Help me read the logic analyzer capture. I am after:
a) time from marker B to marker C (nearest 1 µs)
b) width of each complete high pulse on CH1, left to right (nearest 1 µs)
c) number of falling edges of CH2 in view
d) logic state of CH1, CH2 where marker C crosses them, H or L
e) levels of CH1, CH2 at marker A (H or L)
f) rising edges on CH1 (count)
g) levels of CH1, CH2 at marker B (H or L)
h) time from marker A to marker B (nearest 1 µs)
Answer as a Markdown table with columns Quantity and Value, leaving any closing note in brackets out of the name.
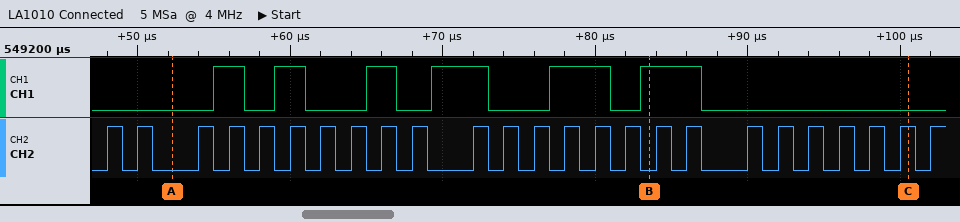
| Quantity | Value |
|---|---|
| time from marker B to marker C | 17 µs |
| width of each complete high pulse on CH1, left to right | 2 µs, 2 µs, 2 µs, 4 µs, 4 µs, 4 µs |
| number of falling edges of CH2 in view | 24 |
| logic state of CH1, CH2 where marker C crosses them, H or L | CH1=L, CH2=H |
| levels of CH1, CH2 at marker A | CH1=L, CH2=L |
| rising edges on CH1 | 6 |
| levels of CH1, CH2 at marker B | CH1=H, CH2=L |
| time from marker A to marker B | 31 µs |
